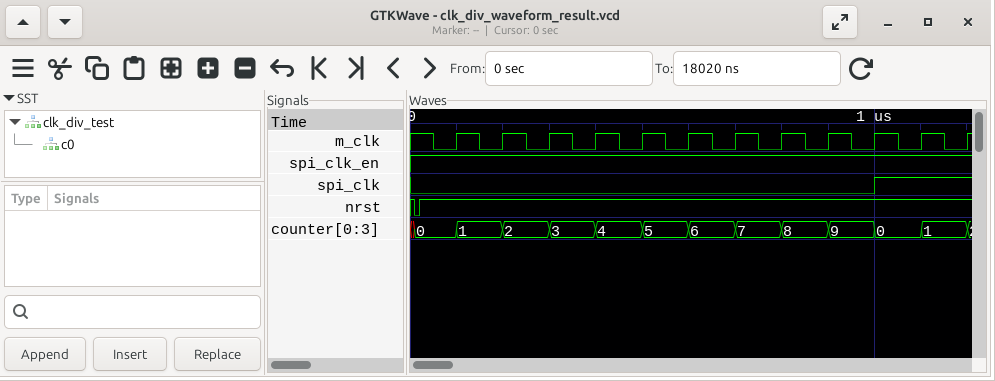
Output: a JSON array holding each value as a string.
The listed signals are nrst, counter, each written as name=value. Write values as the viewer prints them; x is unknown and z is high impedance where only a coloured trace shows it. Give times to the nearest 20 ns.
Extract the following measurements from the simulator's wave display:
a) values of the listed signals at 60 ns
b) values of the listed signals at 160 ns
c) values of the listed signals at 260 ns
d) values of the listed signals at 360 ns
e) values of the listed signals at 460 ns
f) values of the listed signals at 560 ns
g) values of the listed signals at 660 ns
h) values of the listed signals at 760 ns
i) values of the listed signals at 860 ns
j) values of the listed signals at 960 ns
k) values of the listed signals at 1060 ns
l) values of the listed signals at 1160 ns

["nrst=1, counter=0", "nrst=1, counter=1", "nrst=1, counter=2", "nrst=1, counter=3", "nrst=1, counter=4", "nrst=1, counter=5", "nrst=1, counter=6", "nrst=1, counter=7", "nrst=1, counter=8", "nrst=1, counter=9", "nrst=1, counter=0", "nrst=1, counter=1"]
